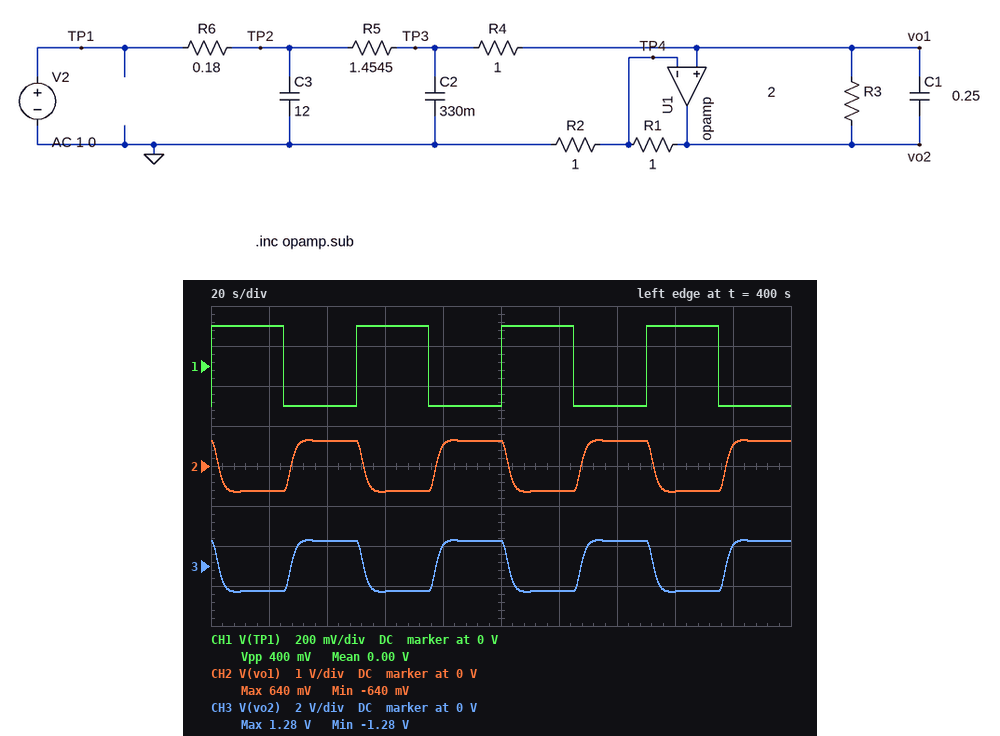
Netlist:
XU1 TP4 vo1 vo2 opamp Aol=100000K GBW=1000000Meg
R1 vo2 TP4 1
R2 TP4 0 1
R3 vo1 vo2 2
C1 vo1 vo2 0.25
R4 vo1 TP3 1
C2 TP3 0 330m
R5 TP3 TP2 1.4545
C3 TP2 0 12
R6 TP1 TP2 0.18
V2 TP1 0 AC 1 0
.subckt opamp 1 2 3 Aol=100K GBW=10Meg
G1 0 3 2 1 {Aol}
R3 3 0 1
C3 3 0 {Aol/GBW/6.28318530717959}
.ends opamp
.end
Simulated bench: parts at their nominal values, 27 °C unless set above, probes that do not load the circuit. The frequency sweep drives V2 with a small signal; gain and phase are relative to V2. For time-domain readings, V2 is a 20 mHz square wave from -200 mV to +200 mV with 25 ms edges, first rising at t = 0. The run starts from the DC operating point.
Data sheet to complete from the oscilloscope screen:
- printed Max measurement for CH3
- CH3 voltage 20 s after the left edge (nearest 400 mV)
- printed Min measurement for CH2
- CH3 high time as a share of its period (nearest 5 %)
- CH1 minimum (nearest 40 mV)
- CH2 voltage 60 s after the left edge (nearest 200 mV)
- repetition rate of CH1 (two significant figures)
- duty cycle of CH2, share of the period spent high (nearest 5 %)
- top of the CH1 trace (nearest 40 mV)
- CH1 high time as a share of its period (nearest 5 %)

1.28 V
-1.2 V
-640 mV
50 %
-200 mV
-600 mV
20 mHz
50 %
200 mV
50 %
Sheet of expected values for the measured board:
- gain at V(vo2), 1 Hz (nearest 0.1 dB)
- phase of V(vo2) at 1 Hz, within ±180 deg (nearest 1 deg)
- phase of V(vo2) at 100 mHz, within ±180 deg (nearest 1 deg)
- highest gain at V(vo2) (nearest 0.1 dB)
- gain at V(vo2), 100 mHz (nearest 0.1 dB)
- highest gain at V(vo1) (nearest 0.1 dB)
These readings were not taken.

-30.8 dB
-58 deg
84 deg
16.0 dB
12.2 dB
10.0 dB
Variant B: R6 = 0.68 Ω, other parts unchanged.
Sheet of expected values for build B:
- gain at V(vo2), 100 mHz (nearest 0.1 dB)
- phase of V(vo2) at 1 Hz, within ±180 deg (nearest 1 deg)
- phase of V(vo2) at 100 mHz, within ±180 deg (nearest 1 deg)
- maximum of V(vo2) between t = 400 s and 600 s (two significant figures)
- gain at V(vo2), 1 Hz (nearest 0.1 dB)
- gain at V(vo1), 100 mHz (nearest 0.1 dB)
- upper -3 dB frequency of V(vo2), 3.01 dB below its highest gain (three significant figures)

3.2 dB
-61 deg
59 deg
710 mV
-42.3 dB
-2.8 dB
58.5 mHz
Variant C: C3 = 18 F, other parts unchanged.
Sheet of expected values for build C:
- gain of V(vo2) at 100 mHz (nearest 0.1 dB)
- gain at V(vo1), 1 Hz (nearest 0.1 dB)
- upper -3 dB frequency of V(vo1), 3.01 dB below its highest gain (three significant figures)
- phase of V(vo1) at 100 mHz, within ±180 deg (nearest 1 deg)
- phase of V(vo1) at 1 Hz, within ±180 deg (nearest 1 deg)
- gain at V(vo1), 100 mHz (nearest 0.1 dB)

9.8 dB
-40.3 dB
66.3 mHz
71 deg
-59 deg
3.8 dB
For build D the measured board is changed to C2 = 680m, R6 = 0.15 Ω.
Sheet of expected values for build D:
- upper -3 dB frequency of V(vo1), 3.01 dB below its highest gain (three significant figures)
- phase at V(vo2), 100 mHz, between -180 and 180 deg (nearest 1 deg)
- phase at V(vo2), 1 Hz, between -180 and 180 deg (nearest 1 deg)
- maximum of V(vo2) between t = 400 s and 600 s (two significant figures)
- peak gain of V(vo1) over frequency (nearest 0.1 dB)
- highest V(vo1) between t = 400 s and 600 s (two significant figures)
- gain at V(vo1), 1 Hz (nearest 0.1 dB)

167 mHz
117 deg
-80 deg
2.1 V
15.6 dB
1.1 V
-40.7 dB
